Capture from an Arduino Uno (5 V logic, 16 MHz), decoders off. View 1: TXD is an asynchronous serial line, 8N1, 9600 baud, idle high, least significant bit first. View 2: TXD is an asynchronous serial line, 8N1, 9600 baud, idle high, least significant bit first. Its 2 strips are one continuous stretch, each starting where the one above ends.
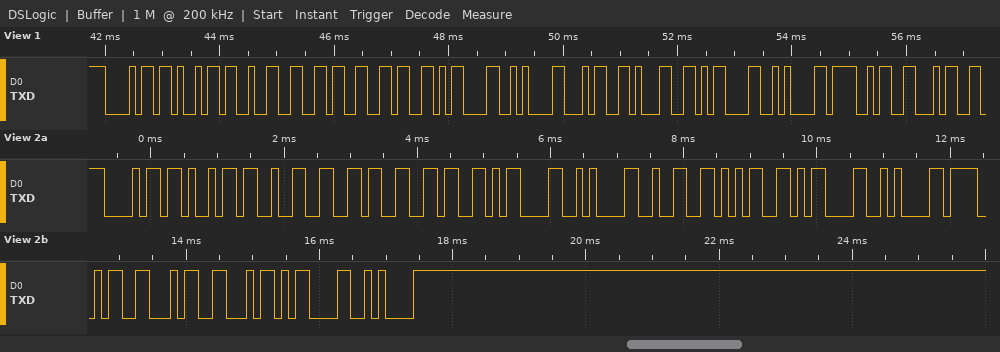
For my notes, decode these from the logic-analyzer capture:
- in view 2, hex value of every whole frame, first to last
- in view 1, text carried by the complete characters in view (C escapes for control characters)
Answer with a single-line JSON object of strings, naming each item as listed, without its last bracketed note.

{"in view 2, hex value of every whole frame, first to last": "0x68 0x69 0x32 0x36 0x36 0x0D 0x0A 0x32 0x35 0x0D 0x0A 0x4F 0x46 0x46 0x0D 0x0A", "in view 1, text carried by the complete characters in view": "\"hi266\\r\\n41\\r\\nOF\""}
